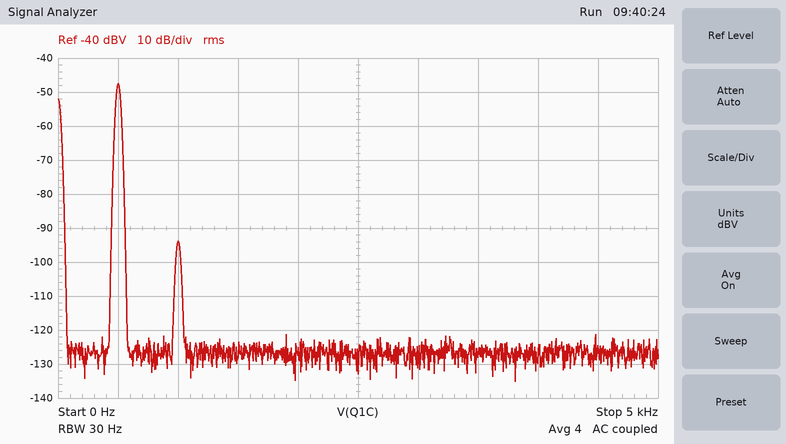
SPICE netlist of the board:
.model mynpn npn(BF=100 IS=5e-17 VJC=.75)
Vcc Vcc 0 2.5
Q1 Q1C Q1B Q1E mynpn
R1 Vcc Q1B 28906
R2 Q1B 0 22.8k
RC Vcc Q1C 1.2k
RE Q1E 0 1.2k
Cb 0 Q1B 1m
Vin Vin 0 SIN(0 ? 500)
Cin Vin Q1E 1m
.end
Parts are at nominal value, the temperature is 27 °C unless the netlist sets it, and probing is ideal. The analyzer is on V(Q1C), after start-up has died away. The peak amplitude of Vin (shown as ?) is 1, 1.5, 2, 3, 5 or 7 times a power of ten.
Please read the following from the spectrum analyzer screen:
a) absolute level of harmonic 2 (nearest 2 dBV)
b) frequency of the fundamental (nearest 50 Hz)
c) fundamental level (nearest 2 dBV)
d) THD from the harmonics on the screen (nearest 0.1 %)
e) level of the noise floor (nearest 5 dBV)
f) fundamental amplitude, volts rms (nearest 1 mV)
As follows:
-94 dBV
500 Hz
-48 dBV
0.5 %
-125 dBV
4 mV
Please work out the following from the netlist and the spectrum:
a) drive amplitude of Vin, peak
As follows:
500 µV
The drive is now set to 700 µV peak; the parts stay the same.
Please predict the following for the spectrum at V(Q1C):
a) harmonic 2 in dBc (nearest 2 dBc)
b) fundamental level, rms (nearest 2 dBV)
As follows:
-44 dBc
-44 dBV
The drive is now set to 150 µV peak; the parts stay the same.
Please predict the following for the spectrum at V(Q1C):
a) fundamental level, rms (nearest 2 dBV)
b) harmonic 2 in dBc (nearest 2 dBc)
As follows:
-58 dBV
-56 dBc
